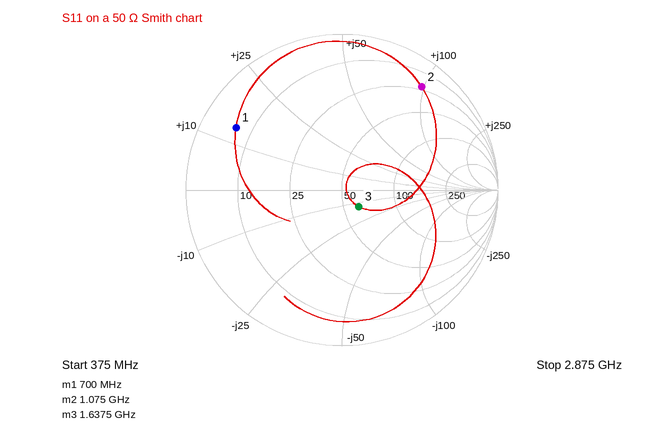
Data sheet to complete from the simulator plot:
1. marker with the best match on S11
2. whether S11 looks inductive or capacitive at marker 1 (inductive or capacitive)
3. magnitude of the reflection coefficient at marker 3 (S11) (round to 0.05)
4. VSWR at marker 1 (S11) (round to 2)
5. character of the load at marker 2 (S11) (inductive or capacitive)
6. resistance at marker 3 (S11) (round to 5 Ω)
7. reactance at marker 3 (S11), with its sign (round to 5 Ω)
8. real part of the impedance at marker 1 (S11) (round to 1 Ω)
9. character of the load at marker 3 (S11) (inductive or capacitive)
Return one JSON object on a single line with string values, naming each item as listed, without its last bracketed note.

{"marker with the best match on S11": "marker 3", "whether S11 looks inductive or capacitive at marker 1": "inductive", "magnitude of the reflection coefficient at marker 3 (S11)": "0.15", "VSWR at marker 1 (S11)": "8", "character of the load at marker 2 (S11)": "inductive", "resistance at marker 3 (S11)": "60 Ω", "reactance at marker 3 (S11), with its sign": "-15 Ω", "real part of the impedance at marker 1 (S11)": "6 Ω", "character of the load at marker 3 (S11)": "capacitive"}
